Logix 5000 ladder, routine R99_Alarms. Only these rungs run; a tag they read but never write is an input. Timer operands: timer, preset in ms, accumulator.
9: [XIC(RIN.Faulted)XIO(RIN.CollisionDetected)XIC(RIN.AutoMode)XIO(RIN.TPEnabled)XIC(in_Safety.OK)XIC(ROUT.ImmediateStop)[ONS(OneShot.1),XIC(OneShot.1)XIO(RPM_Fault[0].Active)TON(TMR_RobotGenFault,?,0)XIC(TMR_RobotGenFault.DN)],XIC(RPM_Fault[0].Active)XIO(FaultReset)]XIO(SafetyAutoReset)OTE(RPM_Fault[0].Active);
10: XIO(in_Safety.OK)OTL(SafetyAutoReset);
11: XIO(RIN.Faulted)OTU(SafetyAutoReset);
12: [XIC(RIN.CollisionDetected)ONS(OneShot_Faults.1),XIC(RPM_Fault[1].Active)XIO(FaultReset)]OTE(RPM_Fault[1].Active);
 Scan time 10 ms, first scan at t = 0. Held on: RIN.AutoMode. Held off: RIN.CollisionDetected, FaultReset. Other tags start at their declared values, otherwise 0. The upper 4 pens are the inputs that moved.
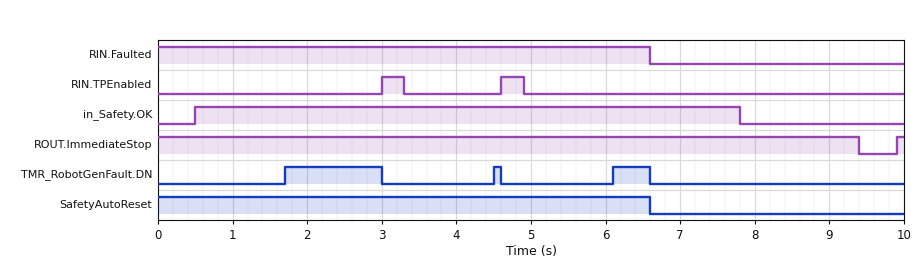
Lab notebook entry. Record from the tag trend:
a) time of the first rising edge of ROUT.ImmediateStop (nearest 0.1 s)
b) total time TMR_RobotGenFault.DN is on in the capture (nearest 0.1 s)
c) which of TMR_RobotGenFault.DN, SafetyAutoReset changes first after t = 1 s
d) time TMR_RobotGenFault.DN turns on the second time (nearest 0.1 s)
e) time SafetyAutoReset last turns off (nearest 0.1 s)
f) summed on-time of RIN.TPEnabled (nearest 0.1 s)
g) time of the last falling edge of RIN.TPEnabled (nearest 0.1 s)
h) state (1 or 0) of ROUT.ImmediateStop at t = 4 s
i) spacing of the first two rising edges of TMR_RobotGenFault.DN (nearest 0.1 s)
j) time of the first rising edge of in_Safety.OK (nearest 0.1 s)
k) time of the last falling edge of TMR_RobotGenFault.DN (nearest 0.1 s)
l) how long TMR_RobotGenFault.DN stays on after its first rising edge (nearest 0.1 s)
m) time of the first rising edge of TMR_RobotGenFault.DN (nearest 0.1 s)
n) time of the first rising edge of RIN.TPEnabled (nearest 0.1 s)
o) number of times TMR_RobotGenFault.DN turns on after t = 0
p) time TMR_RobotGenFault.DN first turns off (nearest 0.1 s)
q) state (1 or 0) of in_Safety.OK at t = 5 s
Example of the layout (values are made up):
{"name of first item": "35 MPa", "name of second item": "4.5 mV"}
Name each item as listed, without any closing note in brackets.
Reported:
{"time of the first rising edge of ROUT.ImmediateStop": "9.9 s", "total time TMR_RobotGenFault.DN is on in the capture": "1.9 s", "which of TMR_RobotGenFault.DN, SafetyAutoReset changes first after t = 1 s": "TMR_RobotGenFault.DN", "time TMR_RobotGenFault.DN turns on the second time": "4.5 s", "time SafetyAutoReset last turns off": "6.6 s", "summed on-time of RIN.TPEnabled": "0.6 s", "time of the last falling edge of RIN.TPEnabled": "4.9 s", "state (1 or 0) of ROUT.ImmediateStop at t = 4 s": "1", "spacing of the first two rising edges of TMR_RobotGenFault.DN": "2.8 s", "time of the first rising edge of in_Safety.OK": "0.5 s", "time of the last falling edge of TMR_RobotGenFault.DN": "6.6 s", "how long TMR_RobotGenFault.DN stays on after its first rising edge": "1.3 s", "time of the first rising edge of TMR_RobotGenFault.DN": "1.7 s", "time of the first rising edge of RIN.TPEnabled": "3.0 s", "number of times TMR_RobotGenFault.DN turns on after t = 0": "3", "time TMR_RobotGenFault.DN first turns off": "3.0 s", "state (1 or 0) of in_Safety.OK at t = 5 s": "1"}
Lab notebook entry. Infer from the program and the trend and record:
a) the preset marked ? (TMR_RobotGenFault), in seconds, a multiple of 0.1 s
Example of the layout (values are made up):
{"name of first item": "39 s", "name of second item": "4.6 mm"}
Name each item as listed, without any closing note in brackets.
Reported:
{"the preset marked ? (TMR_RobotGenFault), in seconds, a multiple of 0.1 s": "1.2 s"}
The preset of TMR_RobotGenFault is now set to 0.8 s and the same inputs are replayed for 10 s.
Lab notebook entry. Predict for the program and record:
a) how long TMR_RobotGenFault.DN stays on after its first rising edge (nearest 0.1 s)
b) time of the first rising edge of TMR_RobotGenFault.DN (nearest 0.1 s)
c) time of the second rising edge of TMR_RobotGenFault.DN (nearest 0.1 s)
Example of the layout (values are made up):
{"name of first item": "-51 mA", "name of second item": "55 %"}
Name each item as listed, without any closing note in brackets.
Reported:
{"how long TMR_RobotGenFault.DN stays on after its first rising edge": "1.7 s", "time of the first rising edge of TMR_RobotGenFault.DN": "1.3 s", "time of the second rising edge of TMR_RobotGenFault.DN": "4.1 s"}
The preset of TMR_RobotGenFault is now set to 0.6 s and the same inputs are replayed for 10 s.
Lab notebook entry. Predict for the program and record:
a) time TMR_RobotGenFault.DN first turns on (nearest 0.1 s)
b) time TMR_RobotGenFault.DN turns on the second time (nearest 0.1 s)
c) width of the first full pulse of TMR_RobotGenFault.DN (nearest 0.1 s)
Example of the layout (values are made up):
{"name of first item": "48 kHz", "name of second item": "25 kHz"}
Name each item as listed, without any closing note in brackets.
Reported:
{"time TMR_RobotGenFault.DN first turns on": "1.1 s", "time TMR_RobotGenFault.DN turns on the second time": "3.9 s", "width of the first full pulse of TMR_RobotGenFault.DN": "1.9 s"}
